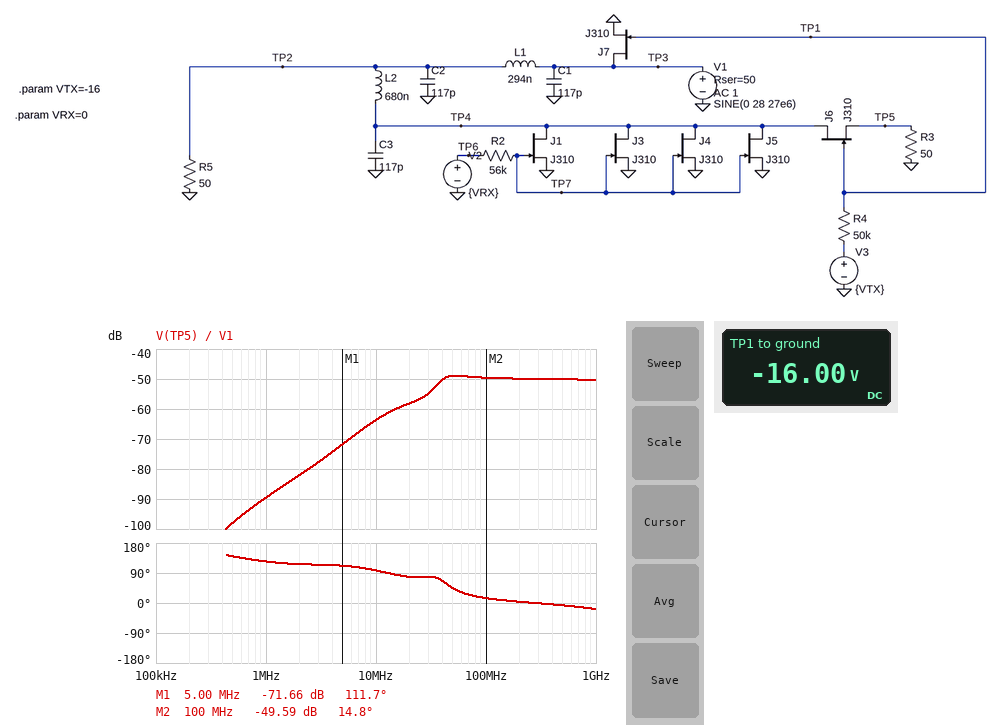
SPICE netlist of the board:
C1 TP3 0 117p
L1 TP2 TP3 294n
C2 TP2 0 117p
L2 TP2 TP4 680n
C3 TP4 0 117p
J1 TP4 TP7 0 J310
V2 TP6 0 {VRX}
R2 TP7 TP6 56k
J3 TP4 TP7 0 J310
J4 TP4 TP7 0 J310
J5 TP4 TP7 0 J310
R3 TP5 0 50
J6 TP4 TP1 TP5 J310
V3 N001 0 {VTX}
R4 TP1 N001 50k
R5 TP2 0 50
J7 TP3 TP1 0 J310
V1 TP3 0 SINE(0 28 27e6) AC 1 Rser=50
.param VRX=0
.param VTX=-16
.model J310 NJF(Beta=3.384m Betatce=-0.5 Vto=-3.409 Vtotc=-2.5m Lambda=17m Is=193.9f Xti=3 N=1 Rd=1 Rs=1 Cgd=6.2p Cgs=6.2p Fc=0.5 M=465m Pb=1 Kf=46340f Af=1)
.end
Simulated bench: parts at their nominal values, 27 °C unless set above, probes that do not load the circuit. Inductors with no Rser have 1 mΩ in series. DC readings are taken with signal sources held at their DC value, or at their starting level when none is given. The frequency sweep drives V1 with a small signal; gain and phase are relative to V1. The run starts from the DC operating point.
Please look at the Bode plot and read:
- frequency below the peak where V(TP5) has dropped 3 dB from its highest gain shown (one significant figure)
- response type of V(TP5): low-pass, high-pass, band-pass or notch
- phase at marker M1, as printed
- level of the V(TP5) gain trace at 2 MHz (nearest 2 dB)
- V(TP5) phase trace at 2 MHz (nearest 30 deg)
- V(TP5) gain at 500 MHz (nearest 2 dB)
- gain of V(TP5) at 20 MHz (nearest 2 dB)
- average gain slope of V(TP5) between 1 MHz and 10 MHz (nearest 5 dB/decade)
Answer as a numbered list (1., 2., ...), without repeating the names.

1. 40 MHz
2. high-pass
3. 111.7 deg
4. -82 dB
5. 120 deg
6. -50 dB
7. -58 dB
8. 25 dB/decade
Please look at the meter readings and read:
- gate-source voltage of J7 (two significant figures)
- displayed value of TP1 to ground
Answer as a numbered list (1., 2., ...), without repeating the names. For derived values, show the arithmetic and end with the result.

1. -16 V = -16 V
2. -16.00 V
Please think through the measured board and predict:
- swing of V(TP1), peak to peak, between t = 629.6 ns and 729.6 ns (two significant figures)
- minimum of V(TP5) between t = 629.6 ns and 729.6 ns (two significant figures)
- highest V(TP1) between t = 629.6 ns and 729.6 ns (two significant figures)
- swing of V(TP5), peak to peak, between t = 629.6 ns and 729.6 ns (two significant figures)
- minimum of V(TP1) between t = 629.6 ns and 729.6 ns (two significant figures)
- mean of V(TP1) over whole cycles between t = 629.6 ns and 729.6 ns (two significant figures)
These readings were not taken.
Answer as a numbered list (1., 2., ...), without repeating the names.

1. 7.3 V
2. -47 mV
3. -13 V
4. 93 mV
5. -20 V
6. -16 V
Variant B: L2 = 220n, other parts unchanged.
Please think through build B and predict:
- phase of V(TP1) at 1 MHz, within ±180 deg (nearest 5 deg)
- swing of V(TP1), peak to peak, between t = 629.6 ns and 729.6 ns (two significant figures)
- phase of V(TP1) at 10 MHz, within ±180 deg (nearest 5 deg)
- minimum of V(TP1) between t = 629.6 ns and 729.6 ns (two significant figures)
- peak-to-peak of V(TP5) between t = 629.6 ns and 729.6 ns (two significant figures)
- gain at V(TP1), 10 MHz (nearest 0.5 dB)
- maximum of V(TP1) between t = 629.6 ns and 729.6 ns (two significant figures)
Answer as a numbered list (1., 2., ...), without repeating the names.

1. 30 deg
2. 9.1 V
3. 20 deg
4. -21 V
5. 120 mV
6. -18.0 dB
7. -12 V
